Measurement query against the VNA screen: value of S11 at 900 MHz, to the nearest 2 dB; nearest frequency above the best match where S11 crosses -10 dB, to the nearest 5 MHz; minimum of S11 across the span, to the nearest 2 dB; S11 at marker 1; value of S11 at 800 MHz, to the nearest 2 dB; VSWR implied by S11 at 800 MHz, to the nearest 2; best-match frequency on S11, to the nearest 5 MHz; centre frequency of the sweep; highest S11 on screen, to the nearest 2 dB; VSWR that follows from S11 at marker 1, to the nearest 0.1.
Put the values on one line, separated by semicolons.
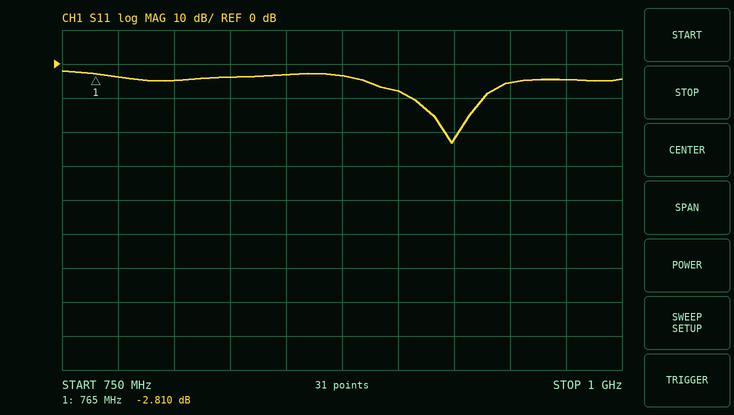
-8 dB; 940 MHz; -24 dB; -2.810 dB; -4 dB; 4; 925 MHz; 875 MHz; -2 dB; 6.2
